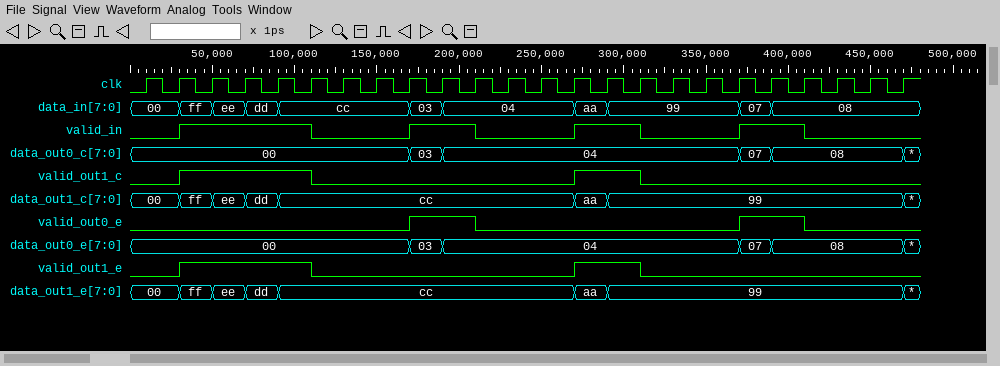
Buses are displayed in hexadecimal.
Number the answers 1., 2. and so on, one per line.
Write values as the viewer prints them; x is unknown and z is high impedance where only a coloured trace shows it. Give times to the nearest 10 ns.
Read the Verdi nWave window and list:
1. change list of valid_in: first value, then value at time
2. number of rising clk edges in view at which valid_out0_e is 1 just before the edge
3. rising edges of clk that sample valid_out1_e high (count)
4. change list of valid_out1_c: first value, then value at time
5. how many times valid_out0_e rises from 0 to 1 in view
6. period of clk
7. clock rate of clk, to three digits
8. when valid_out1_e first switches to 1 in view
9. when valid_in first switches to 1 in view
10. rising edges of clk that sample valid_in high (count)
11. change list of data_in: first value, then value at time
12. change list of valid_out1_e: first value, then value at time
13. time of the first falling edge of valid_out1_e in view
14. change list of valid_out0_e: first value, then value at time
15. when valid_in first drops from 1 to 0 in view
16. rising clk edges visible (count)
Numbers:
1. 0, 1 at 30 ns, 0 at 110 ns, 1 at 170 ns, 0 at 210 ns, 1 at 270 ns, 0 at 310 ns, 1 at 370 ns, 0 at 410 ns
2. 4
3. 6
4. 0, 1 at 30 ns, 0 at 110 ns, 1 at 270 ns, 0 at 310 ns
5. 2
6. 20 ns
7. 50.0 MHz
8. 30 ns
9. 30 ns
10. 10
11. 00, ff at 30 ns, ee at 50 ns, dd at 70 ns, cc at 90 ns, 03 at 170 ns, 04 at 190 ns, aa at 270 ns, 99 at 290 ns, 07 at 370 ns, 08 at 390 ns
12. 0, 1 at 30 ns, 0 at 110 ns, 1 at 270 ns, 0 at 310 ns
13. 110 ns
14. 0, 1 at 170 ns, 0 at 210 ns, 1 at 370 ns, 0 at 410 ns
15. 110 ns
16. 24
